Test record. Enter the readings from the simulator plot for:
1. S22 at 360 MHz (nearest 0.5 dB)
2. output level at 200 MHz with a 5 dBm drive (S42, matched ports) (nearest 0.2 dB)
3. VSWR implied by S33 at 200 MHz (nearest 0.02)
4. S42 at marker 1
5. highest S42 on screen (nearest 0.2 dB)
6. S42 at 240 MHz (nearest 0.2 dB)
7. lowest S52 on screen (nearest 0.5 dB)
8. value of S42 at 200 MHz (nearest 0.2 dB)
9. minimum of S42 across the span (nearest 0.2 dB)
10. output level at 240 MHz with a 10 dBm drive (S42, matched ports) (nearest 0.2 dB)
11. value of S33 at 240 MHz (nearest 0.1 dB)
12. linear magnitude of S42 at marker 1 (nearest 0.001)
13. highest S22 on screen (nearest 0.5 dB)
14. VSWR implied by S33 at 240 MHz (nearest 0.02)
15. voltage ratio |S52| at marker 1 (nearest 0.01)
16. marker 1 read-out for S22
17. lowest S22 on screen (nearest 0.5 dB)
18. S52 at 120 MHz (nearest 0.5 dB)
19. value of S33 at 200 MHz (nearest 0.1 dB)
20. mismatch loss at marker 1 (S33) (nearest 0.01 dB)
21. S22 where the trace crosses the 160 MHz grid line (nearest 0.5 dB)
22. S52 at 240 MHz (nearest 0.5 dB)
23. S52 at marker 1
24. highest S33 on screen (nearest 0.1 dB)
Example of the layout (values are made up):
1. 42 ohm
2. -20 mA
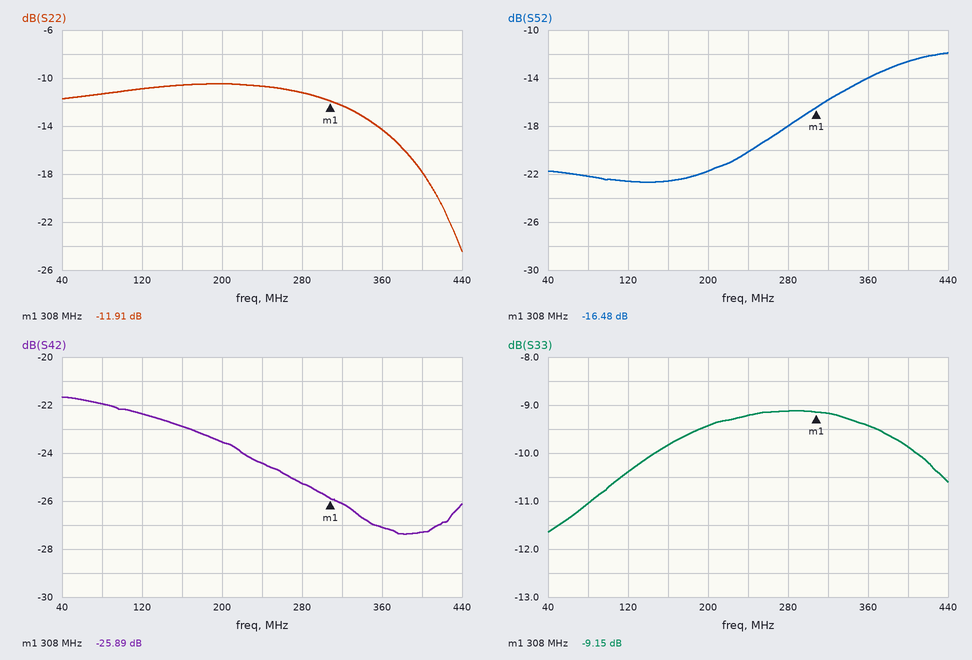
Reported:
1. -14.5 dB
2. -18.6 dBm
3. 2.02
4. -25.89 dB
5. -21.6 dB
6. -24.4 dB
7. -22.5 dB
8. -23.6 dB
9. -27.4 dB
10. -14.4 dBm
11. -9.2 dB
12. 0.051
13. -10.5 dB
14. 2.06
15. 0.15
16. -11.91 dB
17. -24.5 dB
18. -22.5 dB
19. -9.4 dB
20. 0.56 dB
21. -10.5 dB
22. -20.0 dB
23. -16.48 dB
24. -9.1 dB
